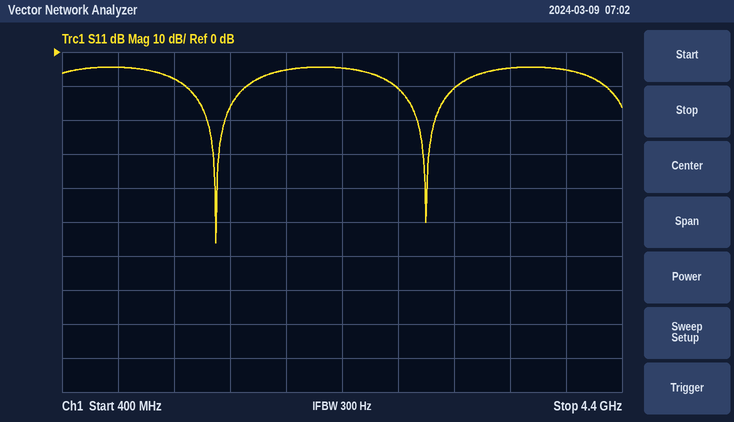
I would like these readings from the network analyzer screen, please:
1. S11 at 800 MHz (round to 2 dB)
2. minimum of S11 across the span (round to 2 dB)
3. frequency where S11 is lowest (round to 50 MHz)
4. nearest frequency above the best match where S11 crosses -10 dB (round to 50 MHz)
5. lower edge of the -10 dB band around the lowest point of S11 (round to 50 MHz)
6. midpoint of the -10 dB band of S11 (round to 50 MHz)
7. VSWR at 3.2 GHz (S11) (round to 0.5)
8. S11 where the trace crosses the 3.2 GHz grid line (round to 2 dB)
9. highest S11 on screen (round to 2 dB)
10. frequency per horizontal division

-4 dB
-56 dB
1.50 GHz
1.70 GHz
1.30 GHz
1.50 GHz
2.0
-10 dB
-4 dB
400 MHz
